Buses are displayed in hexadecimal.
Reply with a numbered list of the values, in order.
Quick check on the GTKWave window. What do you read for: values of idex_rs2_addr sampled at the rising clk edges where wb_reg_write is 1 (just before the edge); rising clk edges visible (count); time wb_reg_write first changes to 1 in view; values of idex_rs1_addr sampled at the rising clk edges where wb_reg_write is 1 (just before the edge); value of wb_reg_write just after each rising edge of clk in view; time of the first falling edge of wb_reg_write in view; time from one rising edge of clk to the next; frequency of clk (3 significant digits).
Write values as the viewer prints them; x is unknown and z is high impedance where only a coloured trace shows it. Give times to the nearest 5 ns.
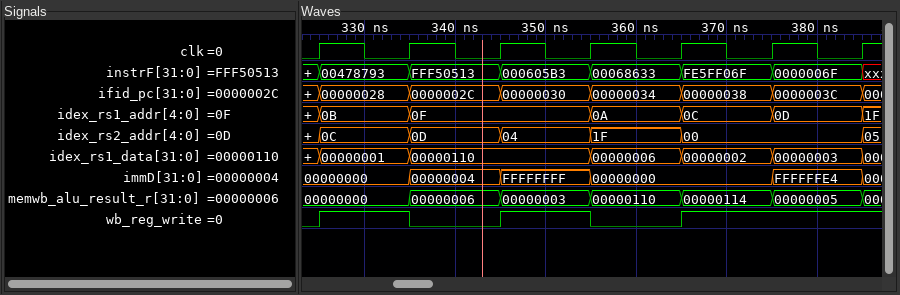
1. 0C, 04, 00, 00
2. 7
3. 325 ns
4. 0B, 0F, 0C, 0D
5. 1 0 1 0 1 1 1
6. 335 ns
7. 10 ns
8. 100 MHz
